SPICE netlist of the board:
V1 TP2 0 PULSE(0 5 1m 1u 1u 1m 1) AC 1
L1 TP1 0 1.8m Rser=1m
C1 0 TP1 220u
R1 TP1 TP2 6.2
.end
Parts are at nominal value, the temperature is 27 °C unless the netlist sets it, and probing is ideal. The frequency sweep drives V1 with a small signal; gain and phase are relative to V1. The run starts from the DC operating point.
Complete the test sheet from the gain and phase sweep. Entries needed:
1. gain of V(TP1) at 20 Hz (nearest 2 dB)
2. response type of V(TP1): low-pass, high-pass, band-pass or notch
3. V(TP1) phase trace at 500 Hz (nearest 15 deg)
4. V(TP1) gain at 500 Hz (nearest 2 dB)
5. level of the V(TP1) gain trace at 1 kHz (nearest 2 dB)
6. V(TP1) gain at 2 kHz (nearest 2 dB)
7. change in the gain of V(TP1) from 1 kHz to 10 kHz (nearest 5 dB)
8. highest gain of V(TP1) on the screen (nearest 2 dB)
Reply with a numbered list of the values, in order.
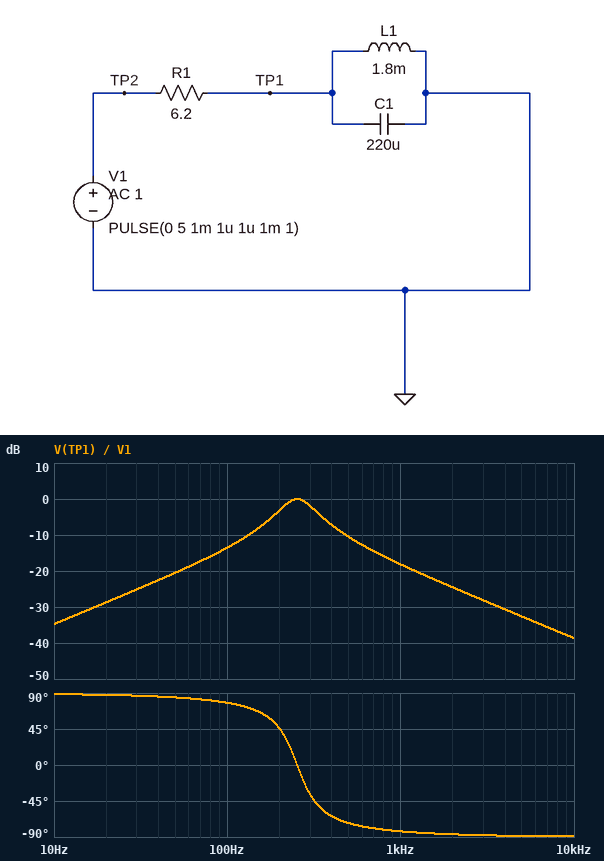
1. -28 dB
2. band-pass
3. -75 deg
4. -10 dB
5. -18 dB
6. -24 dB
7. -20 dB
8. 0 dB
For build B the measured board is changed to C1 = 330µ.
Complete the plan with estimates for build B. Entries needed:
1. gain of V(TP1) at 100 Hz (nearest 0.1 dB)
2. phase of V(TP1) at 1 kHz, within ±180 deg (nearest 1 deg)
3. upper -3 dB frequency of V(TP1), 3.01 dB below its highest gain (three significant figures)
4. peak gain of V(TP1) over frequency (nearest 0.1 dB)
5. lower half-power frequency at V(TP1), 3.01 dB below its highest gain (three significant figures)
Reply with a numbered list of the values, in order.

1. -12.7 dB
2. -85 deg
3. 249 Hz
4. 0 dB
5. 171 Hz
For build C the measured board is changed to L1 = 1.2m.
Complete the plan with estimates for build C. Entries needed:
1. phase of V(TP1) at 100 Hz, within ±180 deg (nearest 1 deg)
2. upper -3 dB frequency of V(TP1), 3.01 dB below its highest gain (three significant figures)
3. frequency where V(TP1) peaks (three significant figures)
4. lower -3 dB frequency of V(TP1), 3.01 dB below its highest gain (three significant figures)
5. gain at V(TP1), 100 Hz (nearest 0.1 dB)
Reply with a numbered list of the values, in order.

1. 82 deg
2. 374 Hz
3. 310 Hz
4. 257 Hz
5. -17.4 dB
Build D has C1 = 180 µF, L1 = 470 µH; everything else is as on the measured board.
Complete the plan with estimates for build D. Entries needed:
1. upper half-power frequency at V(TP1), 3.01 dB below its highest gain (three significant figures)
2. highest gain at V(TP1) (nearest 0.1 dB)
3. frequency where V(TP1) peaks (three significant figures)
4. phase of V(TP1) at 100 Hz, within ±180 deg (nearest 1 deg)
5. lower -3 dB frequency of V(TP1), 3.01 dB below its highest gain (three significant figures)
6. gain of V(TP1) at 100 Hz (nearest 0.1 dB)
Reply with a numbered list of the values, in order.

1. 623 Hz
2. 0 dB
3. 547 Hz
4. 87 deg
5. 480 Hz
6. -26.2 dB
